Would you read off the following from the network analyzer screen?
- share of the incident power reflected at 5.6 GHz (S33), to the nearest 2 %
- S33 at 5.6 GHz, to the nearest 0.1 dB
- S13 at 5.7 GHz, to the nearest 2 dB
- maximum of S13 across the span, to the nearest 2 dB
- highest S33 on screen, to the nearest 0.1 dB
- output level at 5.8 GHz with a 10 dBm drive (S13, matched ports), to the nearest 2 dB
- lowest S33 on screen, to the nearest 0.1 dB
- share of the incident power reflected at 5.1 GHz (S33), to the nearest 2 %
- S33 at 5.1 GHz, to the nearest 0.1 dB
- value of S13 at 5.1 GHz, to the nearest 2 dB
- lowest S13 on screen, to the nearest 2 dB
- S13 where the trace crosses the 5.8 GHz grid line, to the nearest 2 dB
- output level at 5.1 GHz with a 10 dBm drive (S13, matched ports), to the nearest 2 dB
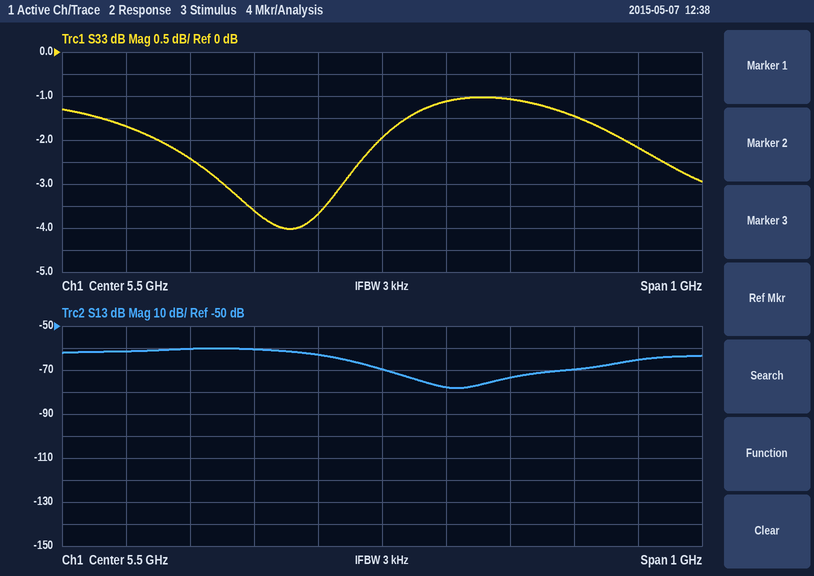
78 %
-1.1 dB
-74 dB
-60 dB
-1.0 dB
-60 dBm
-4.0 dB
68 %
-1.7 dB
-62 dB
-78 dB
-70 dB
-52 dBm
